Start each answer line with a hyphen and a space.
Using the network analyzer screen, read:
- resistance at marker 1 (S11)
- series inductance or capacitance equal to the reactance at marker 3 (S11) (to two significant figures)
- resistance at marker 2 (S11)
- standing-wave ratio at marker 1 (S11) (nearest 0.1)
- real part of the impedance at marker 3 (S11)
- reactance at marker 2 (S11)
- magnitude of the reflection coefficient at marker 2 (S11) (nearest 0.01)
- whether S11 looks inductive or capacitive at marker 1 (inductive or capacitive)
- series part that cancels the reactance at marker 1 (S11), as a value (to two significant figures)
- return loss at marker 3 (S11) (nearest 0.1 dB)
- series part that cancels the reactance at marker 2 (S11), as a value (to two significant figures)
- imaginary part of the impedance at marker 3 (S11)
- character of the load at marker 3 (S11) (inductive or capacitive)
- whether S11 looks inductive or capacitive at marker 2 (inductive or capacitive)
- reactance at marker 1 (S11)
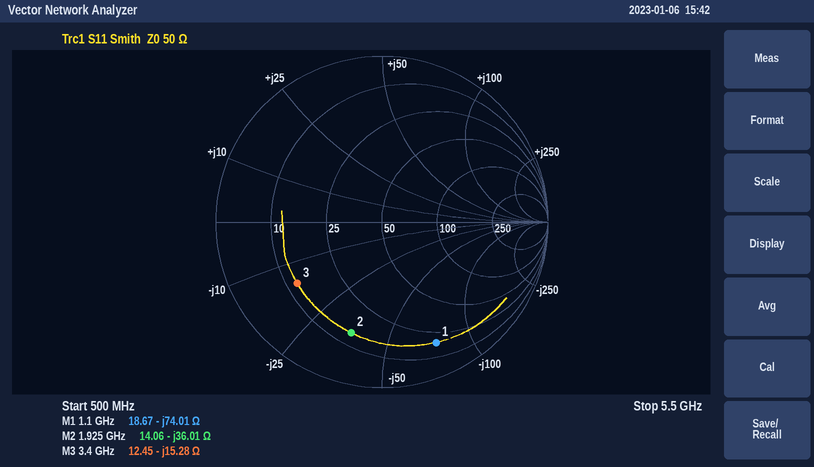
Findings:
- 18.67 Ω
- 3.1 pF
- 14.06 Ω
- 8.8
- 12.45 Ω
- -36.01 Ω
- 0.69
- capacitive
- 11 nH
- 4.0 dB
- 3.0 nH
- -15.28 Ω
- capacitive
- capacitive
- -74.01 Ω
